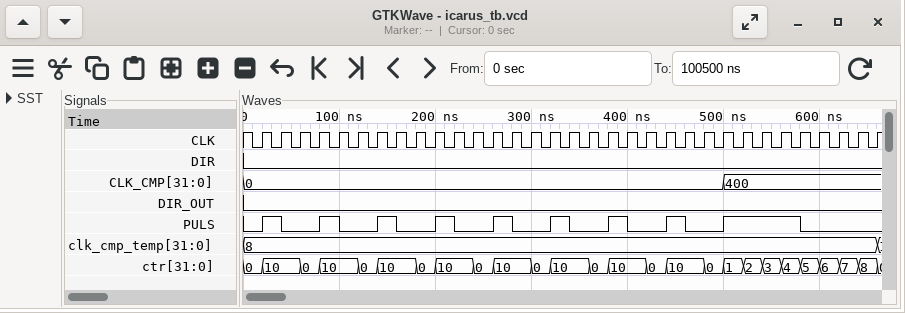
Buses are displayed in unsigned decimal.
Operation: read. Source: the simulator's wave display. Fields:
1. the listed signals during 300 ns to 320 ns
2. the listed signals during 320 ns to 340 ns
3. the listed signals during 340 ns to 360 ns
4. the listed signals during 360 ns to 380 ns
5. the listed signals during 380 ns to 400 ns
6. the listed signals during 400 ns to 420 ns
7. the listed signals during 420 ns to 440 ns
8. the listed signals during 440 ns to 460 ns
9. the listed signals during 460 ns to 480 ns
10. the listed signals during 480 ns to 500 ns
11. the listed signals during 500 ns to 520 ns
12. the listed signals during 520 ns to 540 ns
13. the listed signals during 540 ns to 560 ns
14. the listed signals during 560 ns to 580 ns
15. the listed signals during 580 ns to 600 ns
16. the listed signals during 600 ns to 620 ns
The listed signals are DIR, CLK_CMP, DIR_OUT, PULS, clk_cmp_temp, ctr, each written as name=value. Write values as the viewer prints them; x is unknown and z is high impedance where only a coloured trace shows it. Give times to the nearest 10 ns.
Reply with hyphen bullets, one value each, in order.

- DIR=0, CLK_CMP=0, DIR_OUT=0, PULS=0, clk_cmp_temp=8, ctr=0
- DIR=0, CLK_CMP=0, DIR_OUT=0, PULS=1, clk_cmp_temp=8, ctr=10
- DIR=0, CLK_CMP=0, DIR_OUT=0, PULS=0, clk_cmp_temp=8, ctr=10
- DIR=0, CLK_CMP=0, DIR_OUT=0, PULS=0, clk_cmp_temp=8, ctr=0
- DIR=0, CLK_CMP=0, DIR_OUT=0, PULS=1, clk_cmp_temp=8, ctr=10
- DIR=0, CLK_CMP=0, DIR_OUT=0, PULS=0, clk_cmp_temp=8, ctr=10
- DIR=0, CLK_CMP=0, DIR_OUT=0, PULS=0, clk_cmp_temp=8, ctr=0
- DIR=0, CLK_CMP=0, DIR_OUT=0, PULS=1, clk_cmp_temp=8, ctr=10
- DIR=0, CLK_CMP=0, DIR_OUT=0, PULS=0, clk_cmp_temp=8, ctr=10
- DIR=0, CLK_CMP=0, DIR_OUT=0, PULS=0, clk_cmp_temp=8, ctr=0
- DIR=0, CLK_CMP=400, DIR_OUT=0, PULS=1, clk_cmp_temp=8, ctr=1
- DIR=0, CLK_CMP=400, DIR_OUT=0, PULS=1, clk_cmp_temp=8, ctr=2
- DIR=0, CLK_CMP=400, DIR_OUT=0, PULS=1, clk_cmp_temp=8, ctr=3
- DIR=0, CLK_CMP=400, DIR_OUT=0, PULS=1, clk_cmp_temp=8, ctr=4
- DIR=0, CLK_CMP=400, DIR_OUT=0, PULS=0, clk_cmp_temp=8, ctr=5
- DIR=0, CLK_CMP=400, DIR_OUT=0, PULS=0, clk_cmp_temp=8, ctr=6
